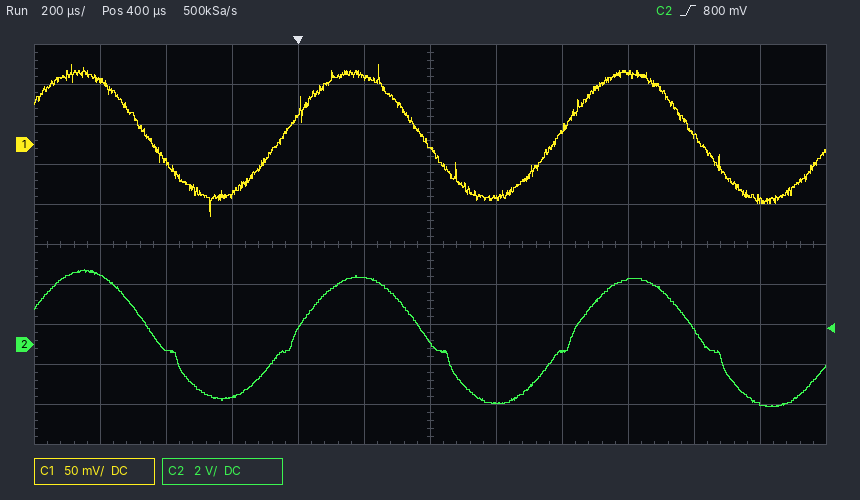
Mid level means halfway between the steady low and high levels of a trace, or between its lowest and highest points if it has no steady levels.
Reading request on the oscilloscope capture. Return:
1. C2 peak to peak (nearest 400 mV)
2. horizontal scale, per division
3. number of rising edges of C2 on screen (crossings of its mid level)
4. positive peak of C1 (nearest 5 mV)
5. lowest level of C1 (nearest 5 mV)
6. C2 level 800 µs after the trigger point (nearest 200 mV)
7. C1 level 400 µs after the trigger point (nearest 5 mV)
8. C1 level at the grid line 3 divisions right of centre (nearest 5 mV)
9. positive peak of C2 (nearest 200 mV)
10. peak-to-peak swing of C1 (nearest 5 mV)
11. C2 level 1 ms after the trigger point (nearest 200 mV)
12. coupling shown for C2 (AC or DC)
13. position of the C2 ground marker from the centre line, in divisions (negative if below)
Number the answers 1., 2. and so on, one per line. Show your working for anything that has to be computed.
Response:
1. 6.8 V
2. 200 µs
3. 2
4. 100 mV
5. -90 mV
6. -400 mV
7. -5 mV
8. 90 mV
9. 3.8 V
10. 100 mV − (-90 mV) = 190 mV
11. 3.2 V
12. DC
13. -2.5 div
